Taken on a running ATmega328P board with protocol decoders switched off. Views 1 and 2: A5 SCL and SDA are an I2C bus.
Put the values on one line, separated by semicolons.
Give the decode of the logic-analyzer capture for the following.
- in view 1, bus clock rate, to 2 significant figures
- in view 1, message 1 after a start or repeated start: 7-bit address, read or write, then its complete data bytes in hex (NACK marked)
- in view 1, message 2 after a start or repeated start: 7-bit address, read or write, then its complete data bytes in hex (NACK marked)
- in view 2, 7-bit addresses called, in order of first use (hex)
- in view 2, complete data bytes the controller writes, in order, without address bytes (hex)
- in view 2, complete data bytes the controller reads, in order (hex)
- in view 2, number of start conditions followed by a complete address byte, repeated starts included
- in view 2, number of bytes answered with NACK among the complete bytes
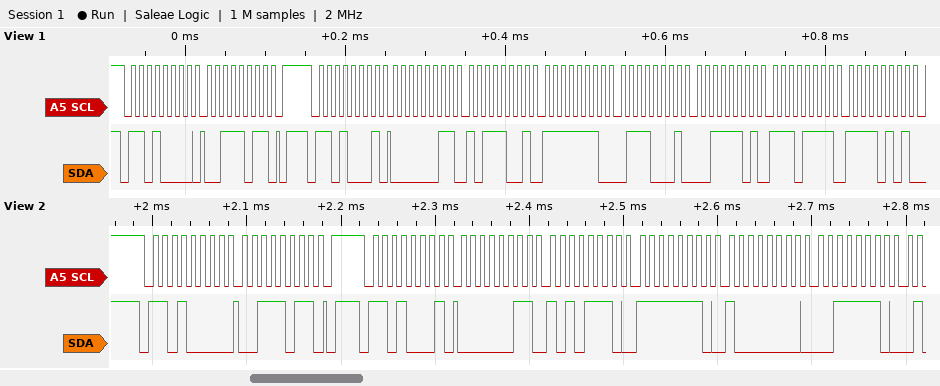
100 kHz; 0x68 write: 3B; 0x68 read: 03 B9 FE 71 3D EF F5; 0x68; 3B; 03 AE FE 80 3E; 2; 0
